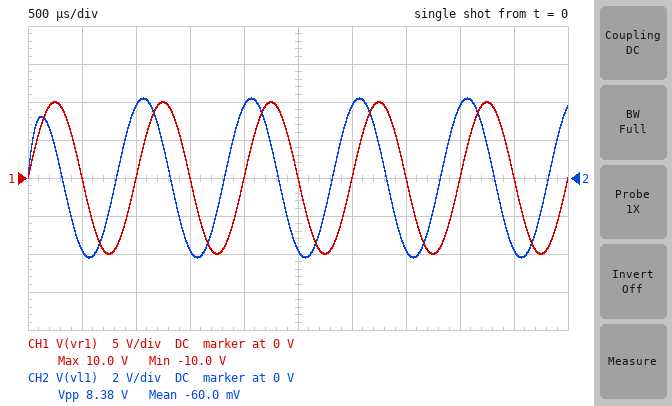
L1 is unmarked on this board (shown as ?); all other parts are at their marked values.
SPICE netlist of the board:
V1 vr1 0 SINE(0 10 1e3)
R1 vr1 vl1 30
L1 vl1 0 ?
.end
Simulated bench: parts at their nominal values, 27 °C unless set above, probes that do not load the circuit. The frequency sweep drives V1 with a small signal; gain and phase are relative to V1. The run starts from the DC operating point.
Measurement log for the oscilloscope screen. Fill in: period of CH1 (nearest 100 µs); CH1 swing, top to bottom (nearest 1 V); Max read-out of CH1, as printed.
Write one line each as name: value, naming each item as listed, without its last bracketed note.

period of CH1: 1.0 ms
CH1 swing, top to bottom: 20 V
Max read-out of CH1, as printed: 10.0 V
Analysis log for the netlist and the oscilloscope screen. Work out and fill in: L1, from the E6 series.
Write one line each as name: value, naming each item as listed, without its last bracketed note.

L1, from the E6 series: 2.2 mH
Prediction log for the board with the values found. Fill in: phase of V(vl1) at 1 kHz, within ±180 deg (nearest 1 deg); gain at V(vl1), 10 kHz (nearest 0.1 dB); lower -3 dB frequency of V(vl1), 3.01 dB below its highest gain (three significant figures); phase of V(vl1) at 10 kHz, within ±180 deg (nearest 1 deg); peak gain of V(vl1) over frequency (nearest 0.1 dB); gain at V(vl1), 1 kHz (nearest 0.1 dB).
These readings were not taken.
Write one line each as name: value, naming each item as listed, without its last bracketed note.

phase of V(vl1) at 1 kHz, within ±180 deg: 65 deg
gain at V(vl1), 10 kHz: -0.2 dB
lower -3 dB frequency of V(vl1), 3.01 dB below its highest gain: 2.17 kHz
phase of V(vl1) at 10 kHz, within ±180 deg: 12 deg
peak gain of V(vl1) over frequency: 0 dB
gain at V(vl1), 1 kHz: -7.6 dB
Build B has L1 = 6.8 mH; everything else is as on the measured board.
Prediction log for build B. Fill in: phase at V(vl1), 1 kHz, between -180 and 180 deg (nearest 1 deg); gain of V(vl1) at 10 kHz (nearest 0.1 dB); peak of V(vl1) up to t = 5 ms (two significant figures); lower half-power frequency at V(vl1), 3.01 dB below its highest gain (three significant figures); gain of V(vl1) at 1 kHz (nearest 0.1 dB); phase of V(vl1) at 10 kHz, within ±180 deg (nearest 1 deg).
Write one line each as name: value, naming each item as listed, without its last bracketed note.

phase at V(vl1), 1 kHz, between -180 and 180 deg: 35 deg
gain of V(vl1) at 10 kHz: 0 dB
peak of V(vl1) up to t = 5 ms: 8.2 V
lower half-power frequency at V(vl1), 3.01 dB below its highest gain: 702 Hz
gain of V(vl1) at 1 kHz: -1.7 dB
phase of V(vl1) at 10 kHz, within ±180 deg: 4 deg
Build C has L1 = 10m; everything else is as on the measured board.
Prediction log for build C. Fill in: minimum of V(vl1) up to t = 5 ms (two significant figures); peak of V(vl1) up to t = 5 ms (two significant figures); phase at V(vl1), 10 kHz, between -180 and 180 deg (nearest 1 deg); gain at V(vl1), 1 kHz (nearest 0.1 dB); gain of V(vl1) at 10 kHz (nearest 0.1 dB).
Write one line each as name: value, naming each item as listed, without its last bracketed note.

minimum of V(vl1) up to t = 5 ms: -9.5 V
peak of V(vl1) up to t = 5 ms: 9.0 V
phase at V(vl1), 10 kHz, between -180 and 180 deg: 3 deg
gain at V(vl1), 1 kHz: -0.9 dB
gain of V(vl1) at 10 kHz: 0 dB
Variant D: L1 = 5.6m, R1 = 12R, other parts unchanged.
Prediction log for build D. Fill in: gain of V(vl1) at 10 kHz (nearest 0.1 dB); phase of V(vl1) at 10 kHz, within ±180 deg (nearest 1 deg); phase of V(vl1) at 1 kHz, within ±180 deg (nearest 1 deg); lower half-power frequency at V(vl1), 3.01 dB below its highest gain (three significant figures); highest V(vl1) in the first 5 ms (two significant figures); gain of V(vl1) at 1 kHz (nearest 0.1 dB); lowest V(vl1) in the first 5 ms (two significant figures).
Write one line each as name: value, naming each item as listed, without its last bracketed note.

gain of V(vl1) at 10 kHz: 0 dB
phase of V(vl1) at 10 kHz, within ±180 deg: 2 deg
phase of V(vl1) at 1 kHz, within ±180 deg: 19 deg
lower half-power frequency at V(vl1), 3.01 dB below its highest gain: 341 Hz
highest V(vl1) in the first 5 ms: 9.5 V
gain of V(vl1) at 1 kHz: -0.5 dB
lowest V(vl1) in the first 5 ms: -10 V
